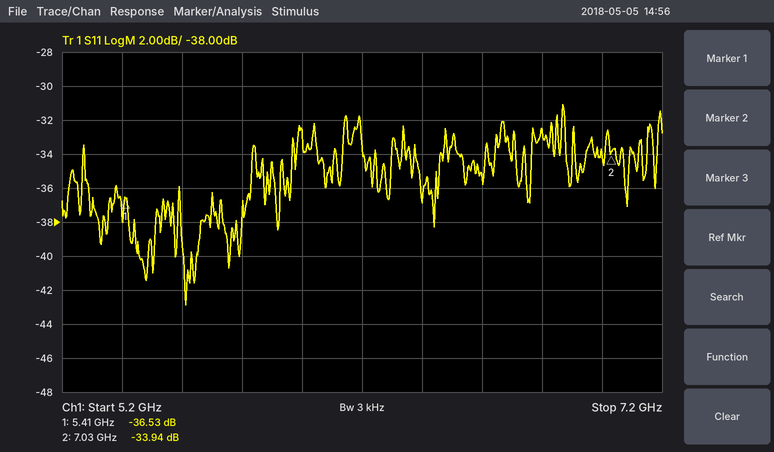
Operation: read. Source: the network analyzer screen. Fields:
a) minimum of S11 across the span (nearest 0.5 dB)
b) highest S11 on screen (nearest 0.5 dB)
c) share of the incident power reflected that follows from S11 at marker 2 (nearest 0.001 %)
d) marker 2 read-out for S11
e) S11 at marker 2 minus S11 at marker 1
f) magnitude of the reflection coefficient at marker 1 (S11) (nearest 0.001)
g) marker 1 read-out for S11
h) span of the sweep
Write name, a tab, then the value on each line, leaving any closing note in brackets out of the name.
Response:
minimum of S11 across the span	-43.0 dB
highest S11 on screen	-31.0 dB
share of the incident power reflected that follows from S11 at marker 2	0.040 %
marker 2 read-out for S11	-33.94 dB
S11 at marker 2 minus S11 at marker 1	2.59 dB
magnitude of the reflection coefficient at marker 1 (S11)	0.015
marker 1 read-out for S11	-36.53 dB
span of the sweep	2 GHz
